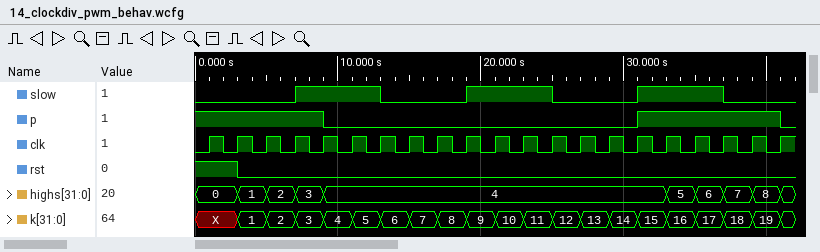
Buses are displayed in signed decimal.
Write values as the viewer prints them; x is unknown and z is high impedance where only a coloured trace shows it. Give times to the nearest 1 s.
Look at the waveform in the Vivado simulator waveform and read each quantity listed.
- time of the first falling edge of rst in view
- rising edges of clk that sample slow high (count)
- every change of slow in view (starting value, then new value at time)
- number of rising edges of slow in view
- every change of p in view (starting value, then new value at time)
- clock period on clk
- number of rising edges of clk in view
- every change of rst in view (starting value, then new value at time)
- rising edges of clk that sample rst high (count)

3 s
9
0, 1 at 7 s, 0 at 13 s, 1 at 19 s, 0 at 25 s, 1 at 31 s, 0 at 37 s
3
1, 0 at 9 s, 1 at 31 s, 0 at 41 s
2 s
21
1, 0 at 3 s
2
